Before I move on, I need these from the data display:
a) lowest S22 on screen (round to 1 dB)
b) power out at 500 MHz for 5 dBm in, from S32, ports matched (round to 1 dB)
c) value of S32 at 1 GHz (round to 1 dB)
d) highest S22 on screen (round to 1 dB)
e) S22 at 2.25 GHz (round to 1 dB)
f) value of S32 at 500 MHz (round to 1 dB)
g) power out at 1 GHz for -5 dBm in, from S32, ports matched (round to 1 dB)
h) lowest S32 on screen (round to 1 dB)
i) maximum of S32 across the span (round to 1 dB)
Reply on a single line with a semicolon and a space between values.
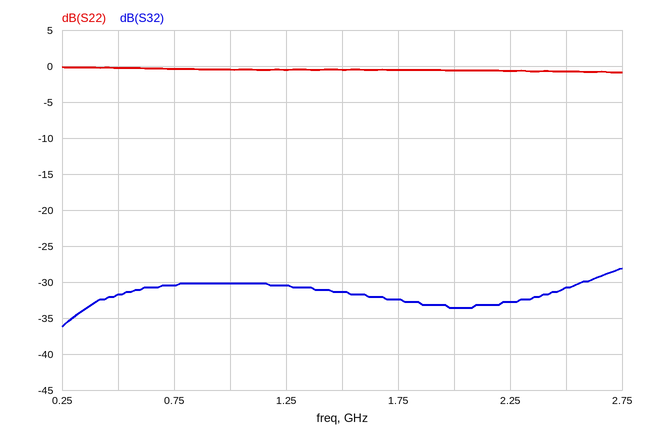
-1 dB; -27 dBm; -30 dB; 0 dB; -1 dB; -32 dB; -35 dBm; -36 dB; -28 dB
